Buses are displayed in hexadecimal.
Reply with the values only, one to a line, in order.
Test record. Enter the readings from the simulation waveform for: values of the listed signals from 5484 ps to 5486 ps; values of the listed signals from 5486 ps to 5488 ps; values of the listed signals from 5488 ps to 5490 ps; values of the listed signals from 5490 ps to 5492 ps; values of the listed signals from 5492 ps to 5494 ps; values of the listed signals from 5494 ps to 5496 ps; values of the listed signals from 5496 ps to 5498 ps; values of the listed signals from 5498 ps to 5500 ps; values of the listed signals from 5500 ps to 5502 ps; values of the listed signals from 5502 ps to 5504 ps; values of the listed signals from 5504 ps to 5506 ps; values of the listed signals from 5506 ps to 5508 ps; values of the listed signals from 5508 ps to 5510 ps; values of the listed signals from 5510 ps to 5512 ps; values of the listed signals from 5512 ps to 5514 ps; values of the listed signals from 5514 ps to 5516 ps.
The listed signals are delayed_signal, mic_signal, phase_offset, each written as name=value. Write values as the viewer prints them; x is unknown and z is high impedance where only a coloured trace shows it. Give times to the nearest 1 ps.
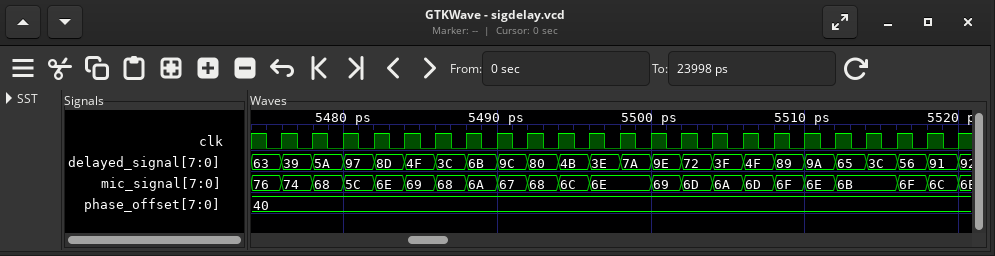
delayed_signal=4F, mic_signal=69, phase_offset=40
delayed_signal=3C, mic_signal=68, phase_offset=40
delayed_signal=6B, mic_signal=6A, phase_offset=40
delayed_signal=9C, mic_signal=67, phase_offset=40
delayed_signal=80, mic_signal=68, phase_offset=40
delayed_signal=4B, mic_signal=6C, phase_offset=40
delayed_signal=3E, mic_signal=6E, phase_offset=40
delayed_signal=7A, mic_signal=6E, phase_offset=40
delayed_signal=9E, mic_signal=69, phase_offset=40
delayed_signal=72, mic_signal=6D, phase_offset=40
delayed_signal=3F, mic_signal=6A, phase_offset=40
delayed_signal=4F, mic_signal=6D, phase_offset=40
delayed_signal=89, mic_signal=6F, phase_offset=40
delayed_signal=9A, mic_signal=6E, phase_offset=40
delayed_signal=65, mic_signal=6B, phase_offset=40
delayed_signal=3C, mic_signal=6B, phase_offset=40
